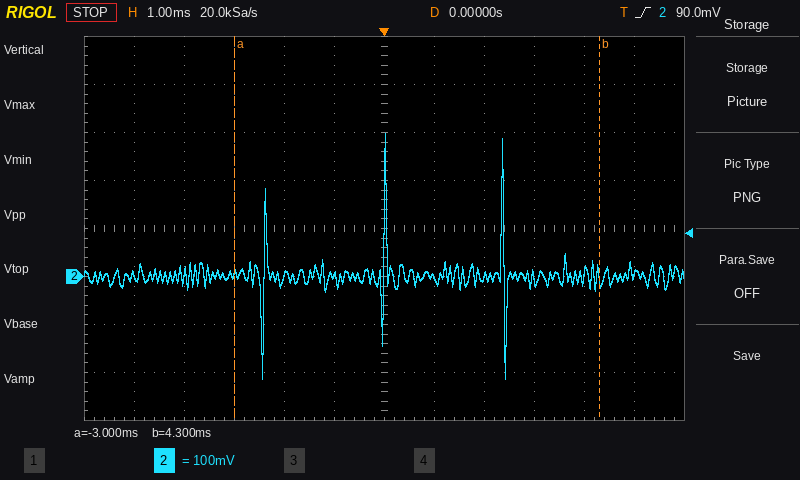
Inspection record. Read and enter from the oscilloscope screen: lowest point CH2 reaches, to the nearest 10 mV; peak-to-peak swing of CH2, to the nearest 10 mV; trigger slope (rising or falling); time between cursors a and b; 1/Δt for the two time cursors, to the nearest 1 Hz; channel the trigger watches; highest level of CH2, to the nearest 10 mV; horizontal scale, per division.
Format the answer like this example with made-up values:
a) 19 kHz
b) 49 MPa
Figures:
a) -210 mV
b) 510 mV
c) rising
d) 7.3 ms
e) 137 Hz
f) CH2
g) 300 mV
h) 1 ms
